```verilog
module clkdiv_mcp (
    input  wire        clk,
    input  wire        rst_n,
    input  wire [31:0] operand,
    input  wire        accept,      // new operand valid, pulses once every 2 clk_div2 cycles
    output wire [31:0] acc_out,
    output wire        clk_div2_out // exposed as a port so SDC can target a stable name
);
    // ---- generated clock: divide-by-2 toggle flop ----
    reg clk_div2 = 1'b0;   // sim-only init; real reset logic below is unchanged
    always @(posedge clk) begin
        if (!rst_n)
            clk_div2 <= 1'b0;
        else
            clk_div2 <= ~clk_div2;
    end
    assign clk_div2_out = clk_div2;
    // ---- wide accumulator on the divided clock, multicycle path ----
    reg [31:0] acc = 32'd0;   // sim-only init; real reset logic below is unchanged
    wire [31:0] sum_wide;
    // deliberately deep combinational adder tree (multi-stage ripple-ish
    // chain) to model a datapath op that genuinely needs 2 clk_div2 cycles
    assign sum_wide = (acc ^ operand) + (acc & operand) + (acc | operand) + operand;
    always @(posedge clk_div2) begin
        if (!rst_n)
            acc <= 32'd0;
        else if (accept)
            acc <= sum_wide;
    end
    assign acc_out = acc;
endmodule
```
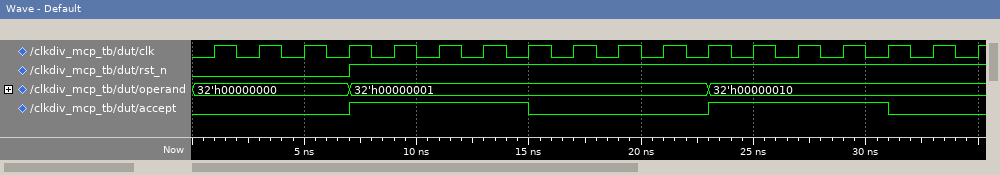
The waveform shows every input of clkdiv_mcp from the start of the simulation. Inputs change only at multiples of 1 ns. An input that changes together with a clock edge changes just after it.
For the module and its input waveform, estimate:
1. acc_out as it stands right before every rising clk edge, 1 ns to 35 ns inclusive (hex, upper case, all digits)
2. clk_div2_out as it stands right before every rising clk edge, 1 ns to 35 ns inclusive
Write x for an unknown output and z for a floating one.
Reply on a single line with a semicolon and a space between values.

00000000, 00000000, 00000000, 00000000, 00000000, 00000003, 00000003, 00000007, 00000007, 00000007, 00000007, 00000007, 00000007, 0000003E, 0000003E, 0000008C, 0000008C, 0000008C; 0 0 0 0 0 1 0 1 0 1 0 1 0 1 0 1 0 1
